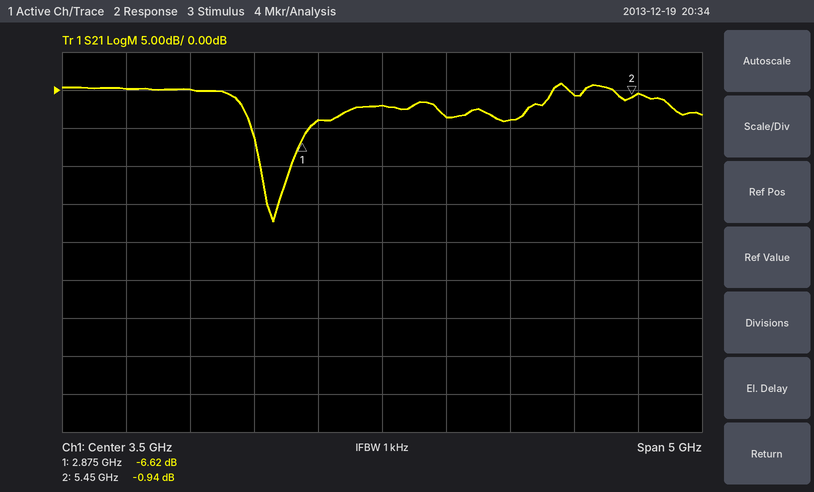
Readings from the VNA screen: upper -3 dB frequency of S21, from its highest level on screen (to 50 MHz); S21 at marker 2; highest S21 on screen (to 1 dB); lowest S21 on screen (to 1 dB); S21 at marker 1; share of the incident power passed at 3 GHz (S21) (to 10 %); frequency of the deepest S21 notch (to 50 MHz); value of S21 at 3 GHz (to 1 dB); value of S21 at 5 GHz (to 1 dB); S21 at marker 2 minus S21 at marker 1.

5.75 GHz
-0.94 dB
1 dB
-17 dB
-6.62 dB
40 %
2.65 GHz
-4 dB
-1 dB
5.68 dB
